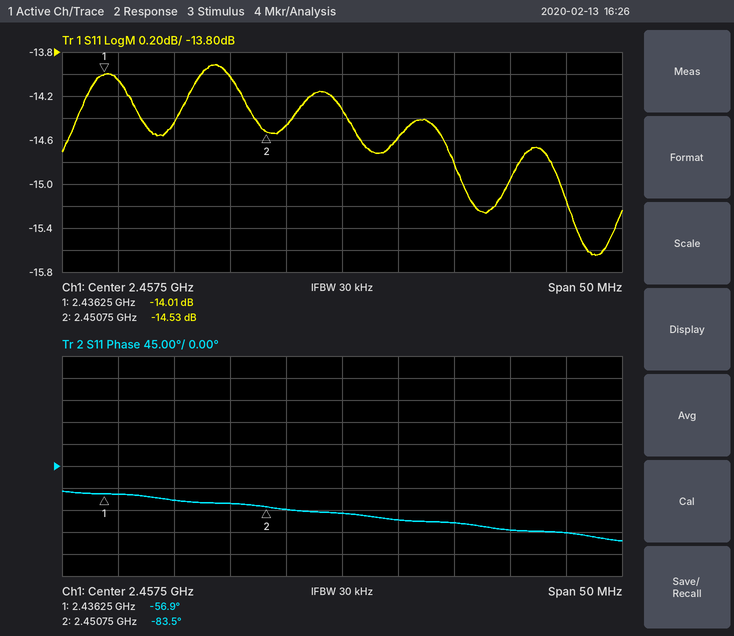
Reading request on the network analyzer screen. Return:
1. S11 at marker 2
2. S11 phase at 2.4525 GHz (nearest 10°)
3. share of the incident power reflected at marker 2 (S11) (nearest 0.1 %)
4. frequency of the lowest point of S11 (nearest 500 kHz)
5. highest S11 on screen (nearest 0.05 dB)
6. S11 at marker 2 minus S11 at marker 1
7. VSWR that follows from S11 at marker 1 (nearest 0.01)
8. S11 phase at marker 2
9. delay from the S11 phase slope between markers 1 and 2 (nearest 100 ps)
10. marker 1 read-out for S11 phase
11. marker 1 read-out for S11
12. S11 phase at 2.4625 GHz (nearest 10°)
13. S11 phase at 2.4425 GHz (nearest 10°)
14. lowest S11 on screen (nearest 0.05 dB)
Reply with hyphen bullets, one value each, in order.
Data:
- -14.53 dB
- -90°
- 3.5 %
- 2.4800 GHz
- -13.90 dB
- -0.52 dB
- 1.50
- -83.5°
- 5.1 ns
- -56.9°
- -14.01 dB
- -110°
- -70°
- -15.65 dB
